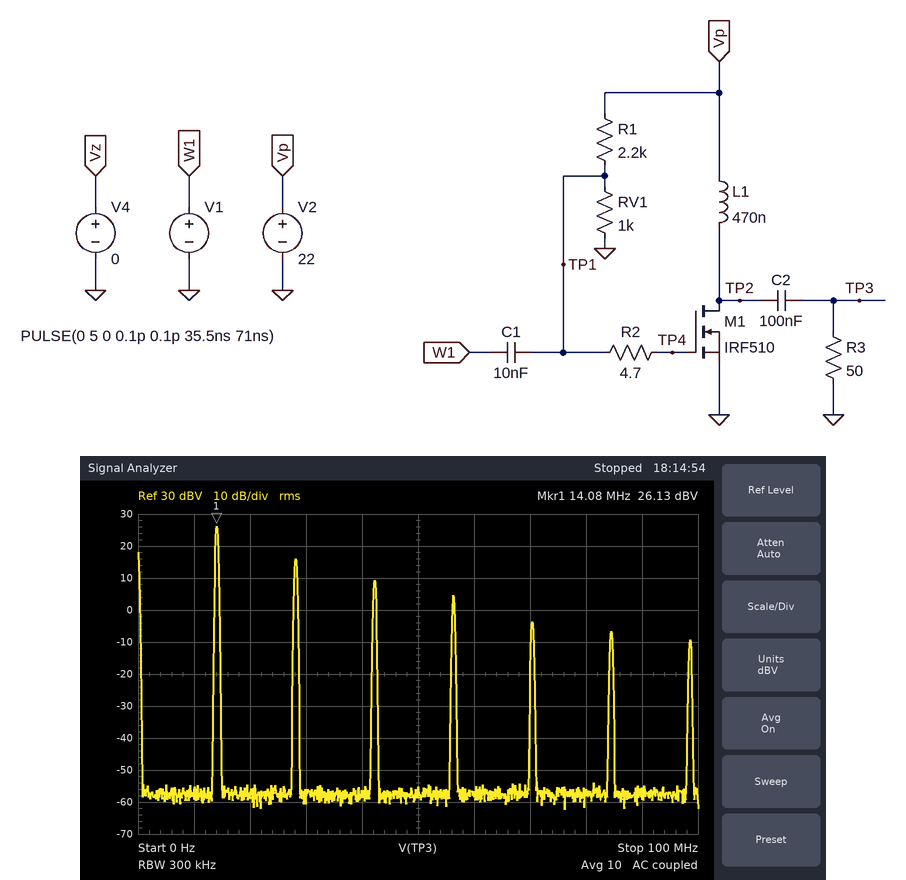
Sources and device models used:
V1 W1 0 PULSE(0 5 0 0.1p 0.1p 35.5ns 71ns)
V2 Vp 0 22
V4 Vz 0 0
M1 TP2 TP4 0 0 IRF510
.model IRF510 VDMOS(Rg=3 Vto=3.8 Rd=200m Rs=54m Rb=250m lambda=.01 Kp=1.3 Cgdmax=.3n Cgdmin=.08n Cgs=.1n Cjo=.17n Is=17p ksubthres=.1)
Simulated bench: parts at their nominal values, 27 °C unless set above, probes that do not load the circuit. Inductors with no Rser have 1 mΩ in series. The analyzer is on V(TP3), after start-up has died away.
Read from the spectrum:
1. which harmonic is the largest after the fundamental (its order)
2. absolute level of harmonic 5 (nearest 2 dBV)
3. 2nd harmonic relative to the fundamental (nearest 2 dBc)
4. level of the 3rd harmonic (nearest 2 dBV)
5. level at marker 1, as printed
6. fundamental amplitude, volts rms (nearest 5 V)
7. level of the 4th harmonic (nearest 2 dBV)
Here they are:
2
-4 dBV
-10 dBc
10 dBV
26.13 dBV
20 V
4 dBV
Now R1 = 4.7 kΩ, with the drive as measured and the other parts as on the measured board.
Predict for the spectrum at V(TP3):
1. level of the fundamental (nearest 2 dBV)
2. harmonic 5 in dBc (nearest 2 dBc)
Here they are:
26 dBV
-32 dBc
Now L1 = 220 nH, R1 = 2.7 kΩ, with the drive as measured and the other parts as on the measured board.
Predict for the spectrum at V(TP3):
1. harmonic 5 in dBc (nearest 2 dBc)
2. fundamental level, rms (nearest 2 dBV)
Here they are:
-34 dBc
26 dBV
